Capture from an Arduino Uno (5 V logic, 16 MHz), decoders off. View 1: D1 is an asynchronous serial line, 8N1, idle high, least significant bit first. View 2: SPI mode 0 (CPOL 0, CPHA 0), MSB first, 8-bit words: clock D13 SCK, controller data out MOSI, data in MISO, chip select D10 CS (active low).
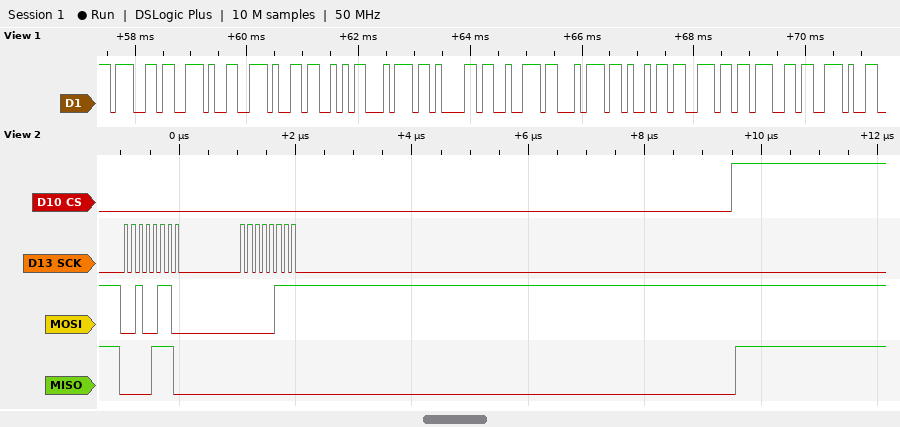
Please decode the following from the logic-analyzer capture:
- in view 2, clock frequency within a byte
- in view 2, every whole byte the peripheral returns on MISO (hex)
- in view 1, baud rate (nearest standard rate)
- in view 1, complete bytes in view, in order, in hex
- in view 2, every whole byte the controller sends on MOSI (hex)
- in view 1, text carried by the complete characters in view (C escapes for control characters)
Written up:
8 MHz
0E 00
9600 baud
67 2E 2E 53 74 61 72 74 69 6E 67 2E
26 07
"g..Starting."
